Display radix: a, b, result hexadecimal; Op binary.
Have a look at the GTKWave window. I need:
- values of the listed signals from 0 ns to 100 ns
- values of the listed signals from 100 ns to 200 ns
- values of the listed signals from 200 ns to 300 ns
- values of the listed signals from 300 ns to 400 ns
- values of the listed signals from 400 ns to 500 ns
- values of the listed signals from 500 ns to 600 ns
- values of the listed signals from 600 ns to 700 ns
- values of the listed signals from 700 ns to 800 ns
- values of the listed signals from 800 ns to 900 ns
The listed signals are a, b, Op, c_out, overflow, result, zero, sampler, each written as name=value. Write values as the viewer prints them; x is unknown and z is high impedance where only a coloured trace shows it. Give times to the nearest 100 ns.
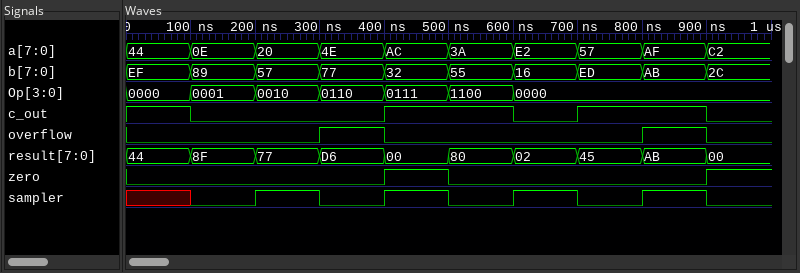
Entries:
a=44, b=EF, Op=0000, c_out=1, overflow=0, result=44, zero=0, sampler=x
a=0E, b=89, Op=0001, c_out=0, overflow=0, result=8F, zero=0, sampler=0
a=20, b=57, Op=0010, c_out=0, overflow=0, result=77, zero=0, sampler=1
a=4E, b=77, Op=0110, c_out=0, overflow=1, result=D6, zero=0, sampler=0
a=AC, b=32, Op=0111, c_out=1, overflow=0, result=00, zero=1, sampler=1
a=3A, b=55, Op=1100, c_out=1, overflow=0, result=80, zero=0, sampler=0
a=E2, b=16, Op=0000, c_out=0, overflow=0, result=02, zero=0, sampler=1
a=57, b=ED, Op=0000, c_out=1, overflow=0, result=45, zero=0, sampler=0
a=AF, b=AB, Op=0000, c_out=1, overflow=1, result=AB, zero=0, sampler=1
